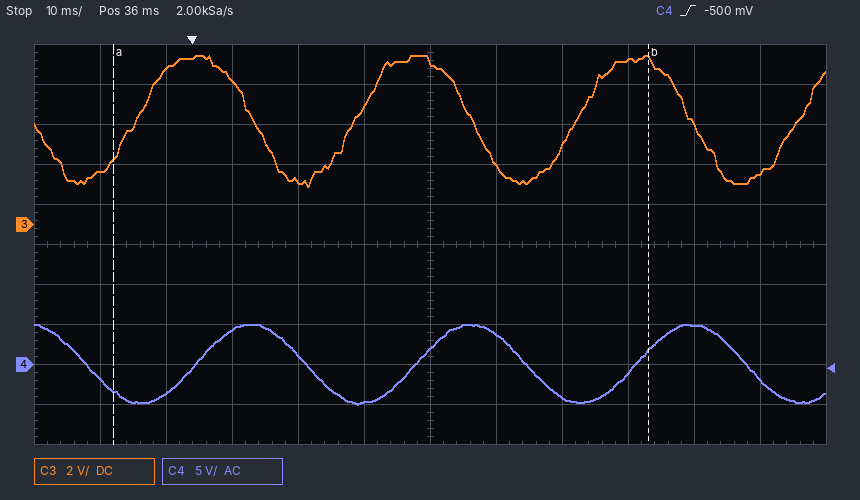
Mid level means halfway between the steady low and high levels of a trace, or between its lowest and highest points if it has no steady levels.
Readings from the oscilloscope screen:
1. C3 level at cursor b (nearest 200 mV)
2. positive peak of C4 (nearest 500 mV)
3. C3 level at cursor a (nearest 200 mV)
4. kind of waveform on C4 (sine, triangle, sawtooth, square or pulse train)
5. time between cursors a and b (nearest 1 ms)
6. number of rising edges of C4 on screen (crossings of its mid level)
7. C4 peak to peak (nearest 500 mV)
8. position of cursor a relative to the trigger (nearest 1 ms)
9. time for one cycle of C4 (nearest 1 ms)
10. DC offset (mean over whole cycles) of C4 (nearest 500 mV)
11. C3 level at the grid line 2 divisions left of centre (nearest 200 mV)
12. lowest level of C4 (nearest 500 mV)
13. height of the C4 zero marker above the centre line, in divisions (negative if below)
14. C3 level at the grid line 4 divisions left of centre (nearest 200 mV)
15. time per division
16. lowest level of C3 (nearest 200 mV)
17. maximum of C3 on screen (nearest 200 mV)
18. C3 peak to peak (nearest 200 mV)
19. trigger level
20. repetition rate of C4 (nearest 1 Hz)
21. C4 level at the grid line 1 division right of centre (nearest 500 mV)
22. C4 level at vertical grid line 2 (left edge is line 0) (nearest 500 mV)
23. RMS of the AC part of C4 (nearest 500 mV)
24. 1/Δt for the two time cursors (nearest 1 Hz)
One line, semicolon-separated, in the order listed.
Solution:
8.2 V; 5.0 V; 3.2 V; sine; 81 ms; 3; 10.0 V; -12 ms; 33 ms; 0.0 V; 2.2 V; -5.0 V; -3.0 div; 7.8 V; 10 ms; 1.8 V; 8.4 V; 6.6 V; -500 mV; 30 Hz; 4.0 V; -3.5 V; 3.5 V; 12 Hz
